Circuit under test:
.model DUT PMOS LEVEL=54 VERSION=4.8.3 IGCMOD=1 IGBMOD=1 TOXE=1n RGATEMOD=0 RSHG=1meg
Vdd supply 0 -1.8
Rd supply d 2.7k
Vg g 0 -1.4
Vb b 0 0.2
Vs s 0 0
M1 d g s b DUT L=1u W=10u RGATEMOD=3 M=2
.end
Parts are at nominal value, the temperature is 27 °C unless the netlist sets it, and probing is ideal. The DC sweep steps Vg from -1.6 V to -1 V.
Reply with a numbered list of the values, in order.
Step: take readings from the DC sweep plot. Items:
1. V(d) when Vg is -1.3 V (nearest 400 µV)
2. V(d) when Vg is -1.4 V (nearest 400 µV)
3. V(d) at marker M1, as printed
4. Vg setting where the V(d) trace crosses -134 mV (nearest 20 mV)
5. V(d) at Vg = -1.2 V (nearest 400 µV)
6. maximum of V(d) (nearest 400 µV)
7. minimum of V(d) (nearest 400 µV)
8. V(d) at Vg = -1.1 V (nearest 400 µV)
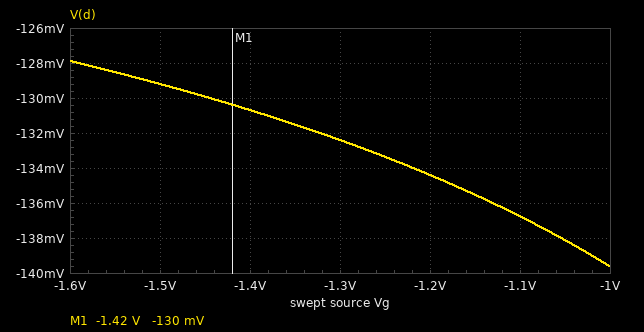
1. -132.4 mV
2. -130.8 mV
3. -130 mV
4. -1.22 V
5. -134.4 mV
6. -128.0 mV
7. -139.6 mV
8. -136.8 mV
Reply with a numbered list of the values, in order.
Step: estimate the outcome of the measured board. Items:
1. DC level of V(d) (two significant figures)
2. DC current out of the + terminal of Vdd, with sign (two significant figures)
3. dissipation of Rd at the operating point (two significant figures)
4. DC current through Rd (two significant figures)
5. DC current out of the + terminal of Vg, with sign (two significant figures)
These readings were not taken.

1. -130 mV
2. -620 µA
3. 1.0 mW
4. 620 µA
5. -520 nA
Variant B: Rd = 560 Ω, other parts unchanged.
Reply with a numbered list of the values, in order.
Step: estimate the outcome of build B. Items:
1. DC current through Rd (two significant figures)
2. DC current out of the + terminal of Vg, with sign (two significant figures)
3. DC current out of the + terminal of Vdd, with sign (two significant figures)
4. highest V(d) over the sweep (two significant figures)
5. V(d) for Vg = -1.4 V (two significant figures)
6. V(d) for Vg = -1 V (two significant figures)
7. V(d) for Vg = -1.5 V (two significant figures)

1. 1.7 mA
2. -500 nA
3. -1.7 mA
4. -790 mV
5. -820 mV
6. -920 mV
7. -810 mV
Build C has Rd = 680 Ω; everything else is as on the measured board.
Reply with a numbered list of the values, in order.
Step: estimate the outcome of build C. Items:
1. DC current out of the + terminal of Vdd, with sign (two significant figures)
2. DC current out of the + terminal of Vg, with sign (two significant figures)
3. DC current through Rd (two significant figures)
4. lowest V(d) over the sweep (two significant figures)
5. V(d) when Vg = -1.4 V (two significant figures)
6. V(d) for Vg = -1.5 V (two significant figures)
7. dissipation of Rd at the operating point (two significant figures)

1. -1.7 mA
2. -500 nA
3. 1.7 mA
4. -750 mV
5. -640 mV
6. -630 mV
7. 2.0 mW
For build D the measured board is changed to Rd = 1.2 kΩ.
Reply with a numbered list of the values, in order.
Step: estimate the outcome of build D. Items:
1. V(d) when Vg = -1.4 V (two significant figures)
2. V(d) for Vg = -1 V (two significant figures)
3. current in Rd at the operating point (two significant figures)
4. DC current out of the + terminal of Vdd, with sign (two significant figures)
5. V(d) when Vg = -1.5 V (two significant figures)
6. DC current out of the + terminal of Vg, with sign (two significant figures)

1. -310 mV
2. -340 mV
3. 1.2 mA
4. -1.2 mA
5. -300 mV
6. -510 nA
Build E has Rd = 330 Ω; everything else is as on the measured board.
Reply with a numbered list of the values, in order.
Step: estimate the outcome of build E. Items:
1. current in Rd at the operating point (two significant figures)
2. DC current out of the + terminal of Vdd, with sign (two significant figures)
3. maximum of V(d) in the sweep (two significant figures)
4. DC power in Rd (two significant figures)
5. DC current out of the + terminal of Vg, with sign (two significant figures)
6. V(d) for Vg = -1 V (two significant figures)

1. 1.8 mA
2. -1.8 mA
3. -1.2 V
4. 1.1 mW
5. -500 nA
6. -1.3 V
